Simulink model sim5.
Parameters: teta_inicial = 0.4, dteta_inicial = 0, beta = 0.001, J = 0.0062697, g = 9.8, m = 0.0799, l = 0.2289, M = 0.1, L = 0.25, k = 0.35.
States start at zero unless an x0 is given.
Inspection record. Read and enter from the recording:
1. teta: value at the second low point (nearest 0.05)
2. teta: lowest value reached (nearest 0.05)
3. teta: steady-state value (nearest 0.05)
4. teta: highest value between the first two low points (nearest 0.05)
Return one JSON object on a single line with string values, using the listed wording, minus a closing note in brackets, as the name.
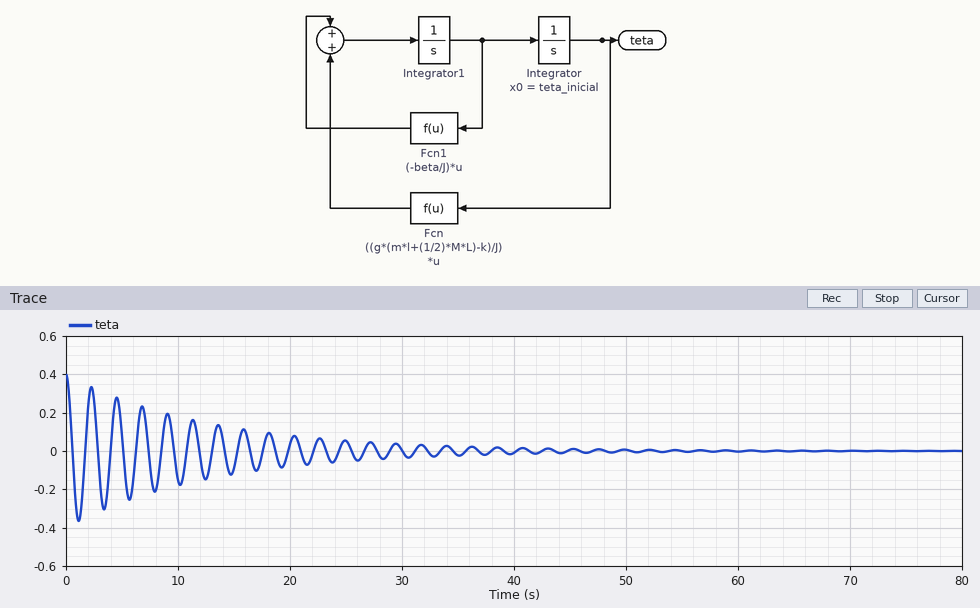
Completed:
{"teta: value at the second low point": "-0.30", "teta: lowest value reached": "-0.35", "teta: steady-state value": "0.00", "teta: highest value between the first two low points": "0.35"}
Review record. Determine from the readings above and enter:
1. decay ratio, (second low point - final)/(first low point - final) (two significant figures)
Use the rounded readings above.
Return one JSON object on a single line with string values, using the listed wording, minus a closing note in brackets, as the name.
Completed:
{"decay ratio, (second low point - final)/(first low point - final)": "0.86"}
